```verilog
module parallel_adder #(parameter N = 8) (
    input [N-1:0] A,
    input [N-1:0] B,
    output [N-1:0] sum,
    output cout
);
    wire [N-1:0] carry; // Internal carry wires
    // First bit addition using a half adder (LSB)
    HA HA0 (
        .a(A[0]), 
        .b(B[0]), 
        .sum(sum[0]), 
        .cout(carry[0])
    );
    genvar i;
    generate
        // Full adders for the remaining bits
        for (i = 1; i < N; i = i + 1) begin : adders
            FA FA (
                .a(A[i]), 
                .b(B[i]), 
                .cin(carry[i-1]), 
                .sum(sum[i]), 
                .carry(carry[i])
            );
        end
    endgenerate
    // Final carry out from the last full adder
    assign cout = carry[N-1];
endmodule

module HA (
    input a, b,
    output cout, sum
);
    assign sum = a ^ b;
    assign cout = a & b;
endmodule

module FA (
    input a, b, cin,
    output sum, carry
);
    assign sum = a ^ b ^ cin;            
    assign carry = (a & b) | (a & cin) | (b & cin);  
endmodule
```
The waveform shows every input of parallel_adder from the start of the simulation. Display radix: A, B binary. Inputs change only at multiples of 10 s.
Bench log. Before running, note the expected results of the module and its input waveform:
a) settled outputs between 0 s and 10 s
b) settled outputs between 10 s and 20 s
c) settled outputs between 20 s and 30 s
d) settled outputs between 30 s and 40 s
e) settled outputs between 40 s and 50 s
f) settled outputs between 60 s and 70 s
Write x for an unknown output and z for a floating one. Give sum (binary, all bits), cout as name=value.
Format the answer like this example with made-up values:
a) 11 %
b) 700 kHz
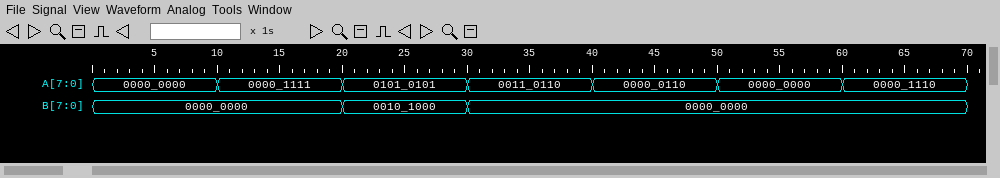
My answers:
a) sum=00000000, cout=0
b) sum=00001111, cout=0
c) sum=01111101, cout=0
d) sum=00110110, cout=0
e) sum=00000110, cout=0
f) sum=00001110, cout=0
